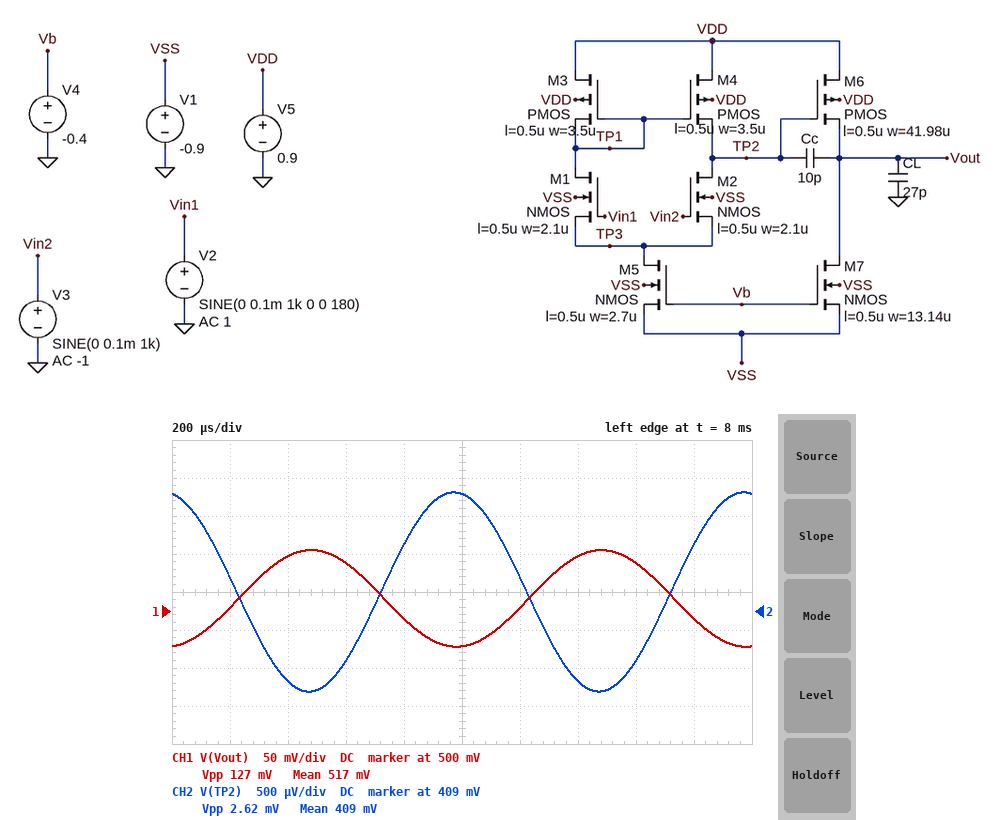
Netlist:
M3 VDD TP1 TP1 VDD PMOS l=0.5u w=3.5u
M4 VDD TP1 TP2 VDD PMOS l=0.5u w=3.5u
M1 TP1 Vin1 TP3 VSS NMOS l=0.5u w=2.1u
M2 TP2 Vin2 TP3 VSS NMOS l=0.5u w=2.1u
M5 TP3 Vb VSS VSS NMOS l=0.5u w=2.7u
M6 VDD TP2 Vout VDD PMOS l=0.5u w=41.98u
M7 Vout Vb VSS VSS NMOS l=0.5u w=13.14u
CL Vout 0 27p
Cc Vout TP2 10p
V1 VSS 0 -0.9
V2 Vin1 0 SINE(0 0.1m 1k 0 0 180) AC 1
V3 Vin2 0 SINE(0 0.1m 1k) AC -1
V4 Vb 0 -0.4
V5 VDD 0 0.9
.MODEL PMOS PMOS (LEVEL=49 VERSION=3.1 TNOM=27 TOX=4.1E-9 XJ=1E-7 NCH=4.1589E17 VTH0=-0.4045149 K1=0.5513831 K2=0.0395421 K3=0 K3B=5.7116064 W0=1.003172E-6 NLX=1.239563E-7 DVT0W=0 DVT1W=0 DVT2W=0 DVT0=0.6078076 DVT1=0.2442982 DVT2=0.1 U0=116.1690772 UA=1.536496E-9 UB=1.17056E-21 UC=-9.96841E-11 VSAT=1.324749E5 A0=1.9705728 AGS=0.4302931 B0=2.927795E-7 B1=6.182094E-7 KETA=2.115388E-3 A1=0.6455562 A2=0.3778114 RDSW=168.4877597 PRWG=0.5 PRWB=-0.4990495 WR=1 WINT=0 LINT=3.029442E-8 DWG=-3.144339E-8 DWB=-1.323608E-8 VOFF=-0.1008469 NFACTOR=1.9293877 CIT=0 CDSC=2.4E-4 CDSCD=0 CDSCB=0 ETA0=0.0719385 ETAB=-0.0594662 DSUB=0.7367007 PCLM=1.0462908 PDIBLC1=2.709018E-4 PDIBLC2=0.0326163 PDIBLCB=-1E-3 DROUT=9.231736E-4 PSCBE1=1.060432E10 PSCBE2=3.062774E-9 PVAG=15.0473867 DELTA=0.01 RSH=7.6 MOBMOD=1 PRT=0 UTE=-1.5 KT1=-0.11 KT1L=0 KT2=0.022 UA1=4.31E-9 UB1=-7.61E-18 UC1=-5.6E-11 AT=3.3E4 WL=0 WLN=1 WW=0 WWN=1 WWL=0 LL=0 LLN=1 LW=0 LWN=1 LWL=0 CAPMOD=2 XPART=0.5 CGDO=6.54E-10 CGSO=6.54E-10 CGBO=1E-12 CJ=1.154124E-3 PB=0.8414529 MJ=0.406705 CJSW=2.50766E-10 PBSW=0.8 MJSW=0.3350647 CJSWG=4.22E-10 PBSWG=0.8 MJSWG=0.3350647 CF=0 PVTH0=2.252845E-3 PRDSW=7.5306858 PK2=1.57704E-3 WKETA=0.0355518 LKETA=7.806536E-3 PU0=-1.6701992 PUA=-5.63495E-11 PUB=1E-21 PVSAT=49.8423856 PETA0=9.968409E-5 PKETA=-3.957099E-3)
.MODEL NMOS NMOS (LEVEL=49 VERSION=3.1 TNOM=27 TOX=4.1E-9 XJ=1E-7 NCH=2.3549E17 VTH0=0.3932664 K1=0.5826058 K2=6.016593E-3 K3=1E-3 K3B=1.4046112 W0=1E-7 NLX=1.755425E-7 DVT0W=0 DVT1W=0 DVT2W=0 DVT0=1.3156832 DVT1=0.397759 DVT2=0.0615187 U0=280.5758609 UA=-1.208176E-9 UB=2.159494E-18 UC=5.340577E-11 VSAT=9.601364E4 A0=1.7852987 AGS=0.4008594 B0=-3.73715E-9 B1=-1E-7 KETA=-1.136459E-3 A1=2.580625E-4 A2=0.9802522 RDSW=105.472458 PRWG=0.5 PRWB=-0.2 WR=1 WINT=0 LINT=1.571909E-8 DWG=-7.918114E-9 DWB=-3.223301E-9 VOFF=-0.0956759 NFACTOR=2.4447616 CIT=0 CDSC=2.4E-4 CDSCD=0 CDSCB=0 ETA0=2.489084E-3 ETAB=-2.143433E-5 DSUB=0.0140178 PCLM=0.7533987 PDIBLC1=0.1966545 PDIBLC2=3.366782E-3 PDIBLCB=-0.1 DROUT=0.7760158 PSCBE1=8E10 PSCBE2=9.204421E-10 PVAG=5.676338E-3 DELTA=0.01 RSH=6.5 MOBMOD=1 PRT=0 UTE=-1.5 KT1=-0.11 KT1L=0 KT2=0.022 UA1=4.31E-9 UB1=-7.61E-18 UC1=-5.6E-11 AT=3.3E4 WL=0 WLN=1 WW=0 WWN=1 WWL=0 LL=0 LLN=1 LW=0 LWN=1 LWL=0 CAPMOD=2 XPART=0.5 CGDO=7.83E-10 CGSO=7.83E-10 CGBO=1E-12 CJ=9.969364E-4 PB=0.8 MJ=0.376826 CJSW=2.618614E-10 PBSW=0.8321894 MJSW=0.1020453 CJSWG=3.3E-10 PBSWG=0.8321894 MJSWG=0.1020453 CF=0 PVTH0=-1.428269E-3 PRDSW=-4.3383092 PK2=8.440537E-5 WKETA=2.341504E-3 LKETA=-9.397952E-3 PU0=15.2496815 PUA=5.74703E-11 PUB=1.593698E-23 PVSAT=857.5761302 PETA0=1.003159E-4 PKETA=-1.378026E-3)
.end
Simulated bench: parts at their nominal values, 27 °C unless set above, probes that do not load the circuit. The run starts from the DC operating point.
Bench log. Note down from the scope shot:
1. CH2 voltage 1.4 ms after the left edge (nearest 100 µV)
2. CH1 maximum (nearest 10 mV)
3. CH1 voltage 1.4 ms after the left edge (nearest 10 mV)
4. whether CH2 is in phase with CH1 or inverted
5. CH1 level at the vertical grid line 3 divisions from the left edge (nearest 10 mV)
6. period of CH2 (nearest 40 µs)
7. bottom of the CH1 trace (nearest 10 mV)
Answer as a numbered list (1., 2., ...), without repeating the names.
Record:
1. 408.1 mV
2. 580 mV
3. 570 mV
4. inverted
5. 560 mV
6. 1.00 ms
7. 450 mV
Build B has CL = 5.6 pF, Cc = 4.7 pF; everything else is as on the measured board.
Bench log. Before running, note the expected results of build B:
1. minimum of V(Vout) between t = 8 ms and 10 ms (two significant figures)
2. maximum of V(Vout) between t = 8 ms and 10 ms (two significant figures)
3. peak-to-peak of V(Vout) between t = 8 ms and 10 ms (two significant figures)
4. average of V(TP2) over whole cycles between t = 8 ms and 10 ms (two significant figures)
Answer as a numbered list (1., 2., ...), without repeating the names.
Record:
1. 380 mV
2. 650 mV
3. 260 mV
4. 410 mV
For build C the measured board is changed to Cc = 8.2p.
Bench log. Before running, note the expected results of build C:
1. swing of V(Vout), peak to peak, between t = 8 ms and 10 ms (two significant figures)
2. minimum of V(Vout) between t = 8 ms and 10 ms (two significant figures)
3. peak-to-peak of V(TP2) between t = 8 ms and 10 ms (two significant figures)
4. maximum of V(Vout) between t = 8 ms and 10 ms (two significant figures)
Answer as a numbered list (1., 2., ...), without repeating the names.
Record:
1. 150 mV
2. 440 mV
3. 3.2 mV
4. 590 mV
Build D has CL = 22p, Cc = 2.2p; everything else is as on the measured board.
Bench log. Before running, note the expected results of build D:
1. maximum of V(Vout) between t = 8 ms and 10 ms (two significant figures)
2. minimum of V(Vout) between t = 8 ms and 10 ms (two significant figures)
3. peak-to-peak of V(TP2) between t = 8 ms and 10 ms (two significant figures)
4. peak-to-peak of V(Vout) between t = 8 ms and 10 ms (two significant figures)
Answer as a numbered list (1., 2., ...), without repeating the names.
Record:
1. 760 mV
2. 260 mV
3. 11 mV
4. 490 mV
